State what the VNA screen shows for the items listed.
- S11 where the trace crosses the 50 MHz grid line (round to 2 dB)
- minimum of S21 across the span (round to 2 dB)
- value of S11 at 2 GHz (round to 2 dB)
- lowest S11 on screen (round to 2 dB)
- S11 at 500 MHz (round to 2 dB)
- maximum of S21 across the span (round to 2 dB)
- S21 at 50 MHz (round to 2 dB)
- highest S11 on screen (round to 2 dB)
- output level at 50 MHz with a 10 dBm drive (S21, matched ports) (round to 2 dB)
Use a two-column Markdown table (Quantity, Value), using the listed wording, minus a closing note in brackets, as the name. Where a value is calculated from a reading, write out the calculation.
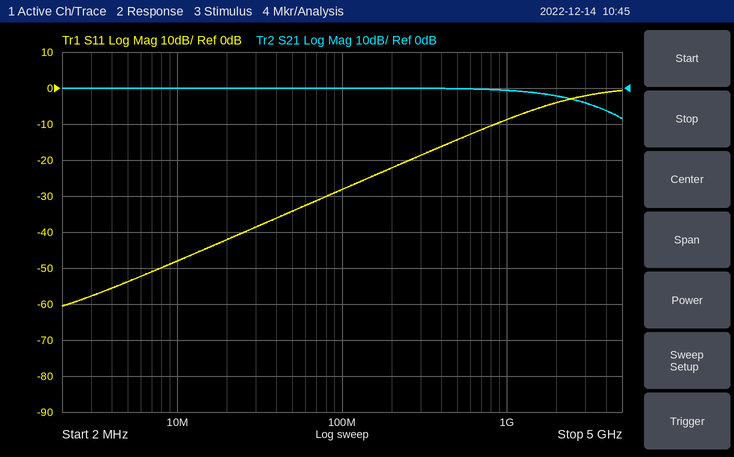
| Quantity | Value |
|---|---|
| S11 where the trace crosses the 50 MHz grid line | -34 dB |
| minimum of S21 across the span | -8 dB |
| value of S11 at 2 GHz | -4 dB |
| lowest S11 on screen | -60 dB |
| S11 at 500 MHz | -14 dB |
| maximum of S21 across the span | 0 dB |
| S21 at 50 MHz | 0 dB |
| highest S11 on screen | 0 dB |
| output level at 50 MHz with a 10 dBm drive (S21, matched ports) | 10 dBm + (0 dB) = 10 dBm |
